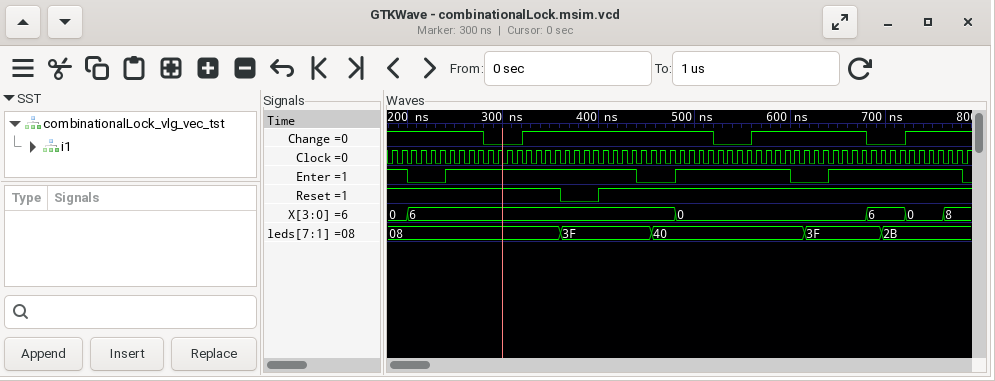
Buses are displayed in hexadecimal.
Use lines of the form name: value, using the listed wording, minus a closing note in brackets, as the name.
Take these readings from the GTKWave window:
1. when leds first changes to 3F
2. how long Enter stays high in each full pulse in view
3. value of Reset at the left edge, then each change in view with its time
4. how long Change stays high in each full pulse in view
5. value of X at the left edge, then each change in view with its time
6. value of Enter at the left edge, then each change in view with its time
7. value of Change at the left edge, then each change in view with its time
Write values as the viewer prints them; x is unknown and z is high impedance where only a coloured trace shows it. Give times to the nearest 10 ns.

when leds first changes to 3F: 360 ns
how long Enter stays high in each full pulse in view: 200 ns, 120 ns, 140 ns
value of Reset at the left edge, then each change in view with its time: 1, 0 at 360 ns, 1 at 400 ns
how long Change stays high in each full pulse in view: 200 ns, 120 ns
value of X at the left edge, then each change in view with its time: 0, 6 at 200 ns, 0 at 480 ns, 6 at 680 ns, 0 at 720 ns, 8 at 760 ns
value of Enter at the left edge, then each change in view with its time: 1, 0 at 200 ns, 1 at 240 ns, 0 at 440 ns, 1 at 480 ns, 0 at 600 ns, 1 at 640 ns, 0 at 780 ns
value of Change at the left edge, then each change in view with its time: 1, 0 at 280 ns, 1 at 320 ns, 0 at 520 ns, 1 at 560 ns, 0 at 680 ns, 1 at 720 ns
